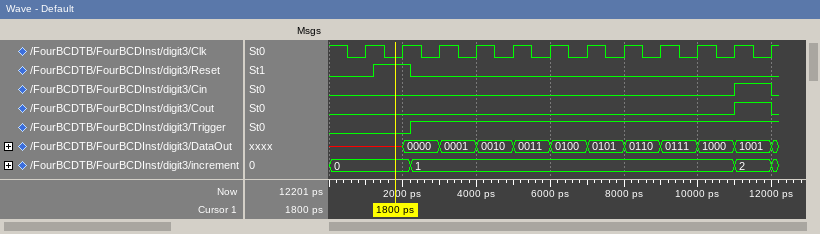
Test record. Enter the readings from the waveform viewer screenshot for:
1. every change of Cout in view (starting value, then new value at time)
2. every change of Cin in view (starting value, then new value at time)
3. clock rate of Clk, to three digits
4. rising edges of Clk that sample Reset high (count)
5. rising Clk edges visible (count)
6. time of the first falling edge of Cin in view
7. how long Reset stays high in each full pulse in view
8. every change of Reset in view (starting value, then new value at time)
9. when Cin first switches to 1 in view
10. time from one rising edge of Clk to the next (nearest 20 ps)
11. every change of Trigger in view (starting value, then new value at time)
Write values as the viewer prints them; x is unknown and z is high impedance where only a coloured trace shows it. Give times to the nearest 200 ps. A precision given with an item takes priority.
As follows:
0, 1 at 11000 ps, 0 at 12000 ps
0, 1 at 11000 ps, 0 at 12000 ps
1.00 GHz
1
12
12000 ps
1000 ps
0, 1 at 1200 ps, 0 at 2200 ps
11000 ps
1000 ps
0, 1 at 2200 ps
